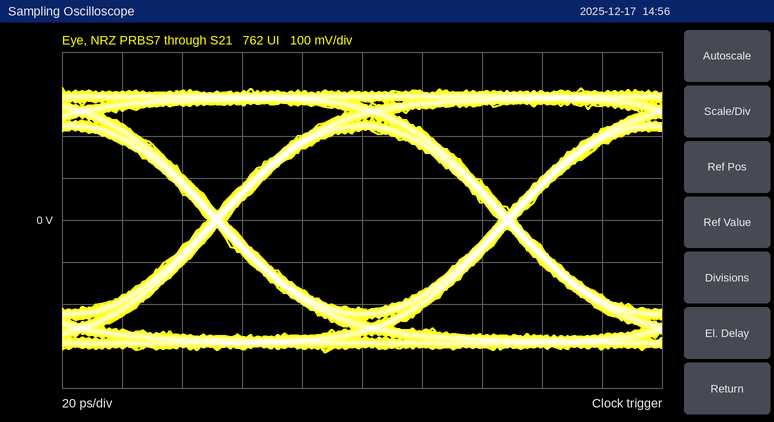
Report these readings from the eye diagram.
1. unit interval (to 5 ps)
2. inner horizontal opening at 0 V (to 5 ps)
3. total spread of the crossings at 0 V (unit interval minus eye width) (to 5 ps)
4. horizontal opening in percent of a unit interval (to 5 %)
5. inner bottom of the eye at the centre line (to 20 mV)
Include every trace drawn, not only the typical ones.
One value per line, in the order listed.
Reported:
95 ps
90 ps
5 ps
95 %
-220 mV
